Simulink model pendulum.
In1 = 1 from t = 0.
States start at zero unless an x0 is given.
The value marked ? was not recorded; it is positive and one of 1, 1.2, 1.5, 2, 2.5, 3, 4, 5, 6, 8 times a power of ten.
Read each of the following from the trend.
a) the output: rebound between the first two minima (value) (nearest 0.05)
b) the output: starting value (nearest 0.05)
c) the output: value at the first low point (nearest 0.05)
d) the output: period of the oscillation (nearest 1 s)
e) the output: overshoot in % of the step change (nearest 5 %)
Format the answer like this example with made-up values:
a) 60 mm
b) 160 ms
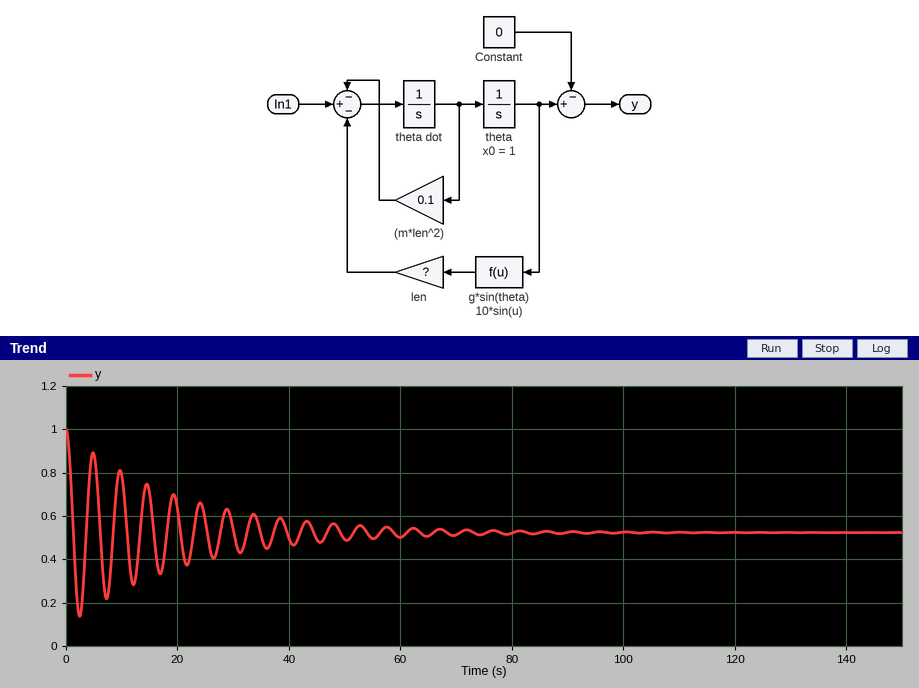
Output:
a) 0.90
b) 1.00
c) 0.15
d) 5 s
e) 80 %
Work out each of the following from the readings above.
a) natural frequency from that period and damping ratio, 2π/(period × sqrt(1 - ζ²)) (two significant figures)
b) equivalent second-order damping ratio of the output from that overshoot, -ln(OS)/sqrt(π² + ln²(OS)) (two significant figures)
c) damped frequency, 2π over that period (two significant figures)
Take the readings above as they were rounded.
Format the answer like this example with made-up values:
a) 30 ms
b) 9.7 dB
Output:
a) 1.3 rad/s
b) 0.071
c) 1.3 rad/s
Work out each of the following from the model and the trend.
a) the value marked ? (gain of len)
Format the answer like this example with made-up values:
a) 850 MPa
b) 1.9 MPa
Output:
a) 0.2
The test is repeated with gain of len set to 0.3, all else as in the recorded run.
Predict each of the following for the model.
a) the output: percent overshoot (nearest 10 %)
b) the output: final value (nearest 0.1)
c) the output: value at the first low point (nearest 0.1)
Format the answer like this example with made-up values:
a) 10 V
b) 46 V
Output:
a) 80 %
b) 0.3
c) -0.2
